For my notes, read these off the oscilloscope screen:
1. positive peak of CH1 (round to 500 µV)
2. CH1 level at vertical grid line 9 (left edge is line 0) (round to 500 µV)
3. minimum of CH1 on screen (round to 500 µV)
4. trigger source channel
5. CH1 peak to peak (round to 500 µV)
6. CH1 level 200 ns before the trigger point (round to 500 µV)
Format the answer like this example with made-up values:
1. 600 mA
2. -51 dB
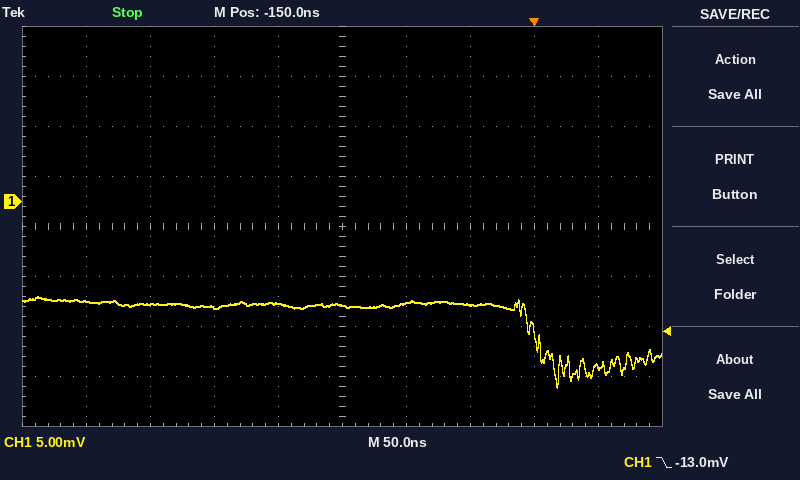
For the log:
1. -9.5 mV
2. -16.5 mV
3. -18.5 mV
4. CH1
5. 9.0 mV
6. -10.0 mV
